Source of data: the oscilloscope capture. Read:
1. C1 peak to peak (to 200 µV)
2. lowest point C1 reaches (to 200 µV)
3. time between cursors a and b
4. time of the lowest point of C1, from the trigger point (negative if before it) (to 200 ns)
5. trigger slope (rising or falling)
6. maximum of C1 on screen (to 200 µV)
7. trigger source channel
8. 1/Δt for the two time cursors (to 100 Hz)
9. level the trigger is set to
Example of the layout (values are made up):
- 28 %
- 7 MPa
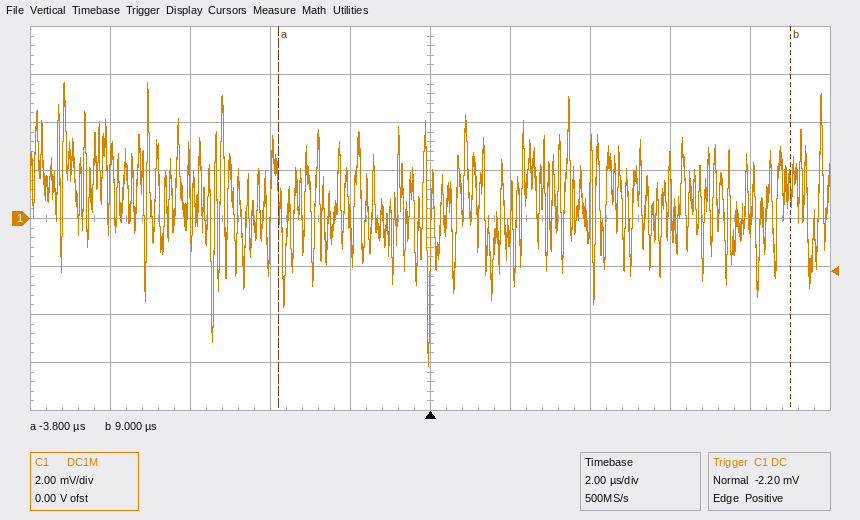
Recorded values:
- 11.8 mV
- -6.2 mV
- 12.8 µs
- 0.0 µs
- rising
- 5.6 mV
- C1
- 78.1 kHz
- -2.20 mV
